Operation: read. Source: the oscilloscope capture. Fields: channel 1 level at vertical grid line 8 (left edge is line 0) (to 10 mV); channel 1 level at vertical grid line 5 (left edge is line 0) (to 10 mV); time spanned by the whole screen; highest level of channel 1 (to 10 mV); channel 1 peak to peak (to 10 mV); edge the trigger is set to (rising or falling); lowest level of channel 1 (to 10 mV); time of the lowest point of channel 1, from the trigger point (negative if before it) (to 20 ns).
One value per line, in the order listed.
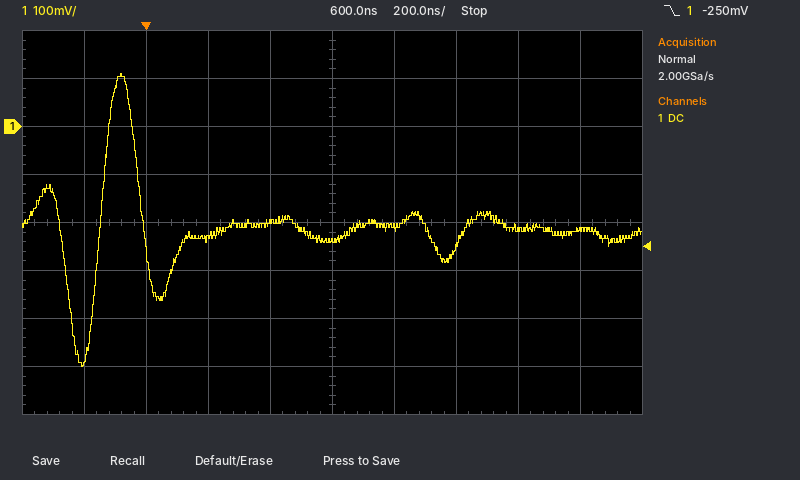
-210 mV
-240 mV
2 µs
110 mV
610 mV
falling
-500 mV
-200 ns
